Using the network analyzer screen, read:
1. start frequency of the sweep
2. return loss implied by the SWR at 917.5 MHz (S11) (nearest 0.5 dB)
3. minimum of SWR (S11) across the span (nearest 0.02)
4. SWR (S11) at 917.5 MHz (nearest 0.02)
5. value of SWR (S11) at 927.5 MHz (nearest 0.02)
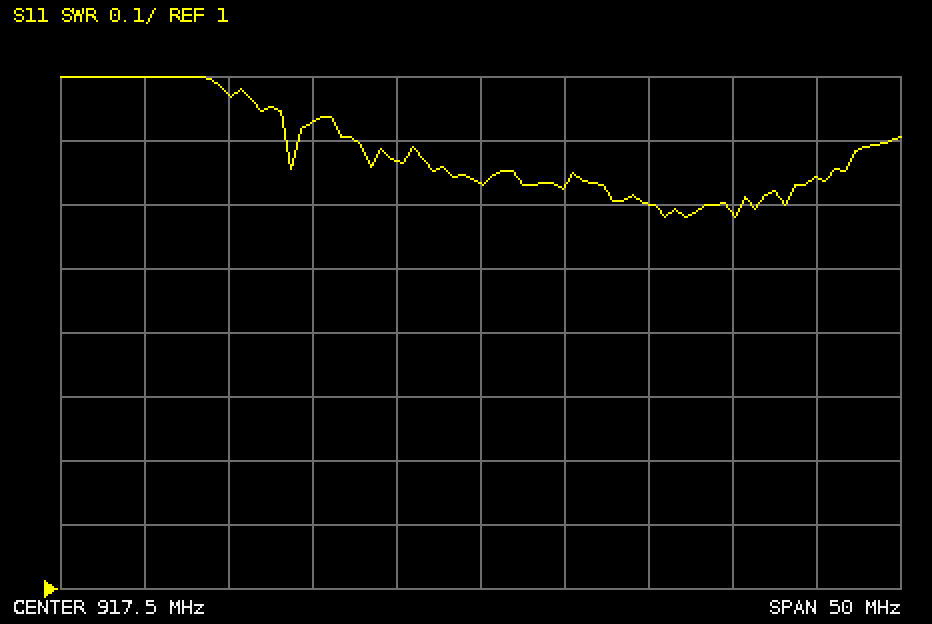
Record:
892.5 MHz
12.5 dB
1.58
1.64
1.60
